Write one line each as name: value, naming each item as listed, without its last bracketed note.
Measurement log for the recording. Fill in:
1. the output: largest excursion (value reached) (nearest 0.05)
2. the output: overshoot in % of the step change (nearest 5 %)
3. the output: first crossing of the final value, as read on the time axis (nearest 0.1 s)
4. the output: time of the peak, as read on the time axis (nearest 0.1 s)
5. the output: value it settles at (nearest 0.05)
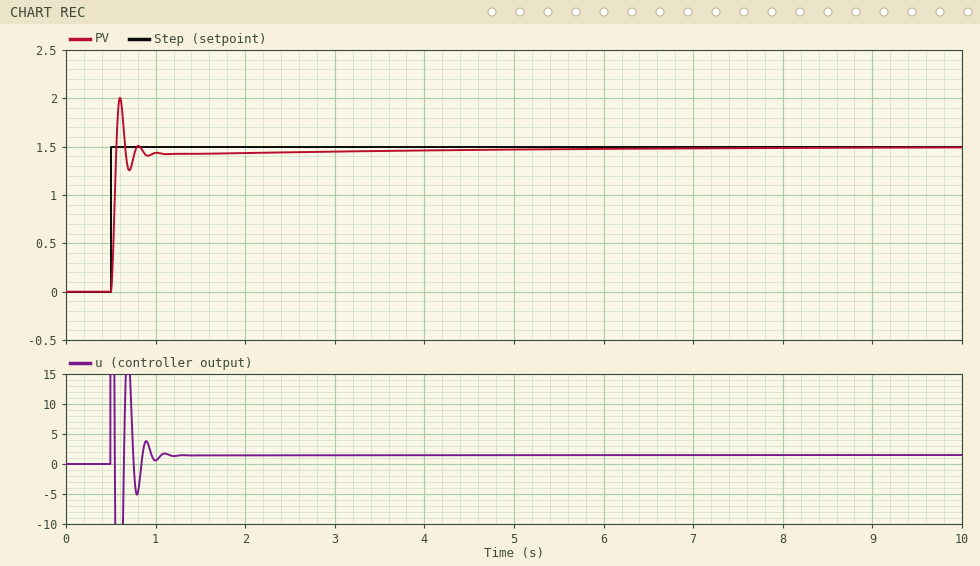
the output: largest excursion (value reached): 2.00
the output: overshoot in % of the step change: 35 %
the output: first crossing of the final value, as read on the time axis: 0.6 s
the output: time of the peak, as read on the time axis: 0.6 s
the output: value it settles at: 1.50
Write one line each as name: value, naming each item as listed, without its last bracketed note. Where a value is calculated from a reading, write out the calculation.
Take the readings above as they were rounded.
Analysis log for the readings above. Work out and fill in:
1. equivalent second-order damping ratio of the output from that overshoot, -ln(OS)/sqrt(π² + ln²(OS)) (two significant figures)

equivalent second-order damping ratio of the output from that overshoot, -ln(OS)/sqrt(π² + ln²(OS)): ln(0.35) = -1.050; 1.050 / sqrt(9.870 + 1.102) = 0.32
